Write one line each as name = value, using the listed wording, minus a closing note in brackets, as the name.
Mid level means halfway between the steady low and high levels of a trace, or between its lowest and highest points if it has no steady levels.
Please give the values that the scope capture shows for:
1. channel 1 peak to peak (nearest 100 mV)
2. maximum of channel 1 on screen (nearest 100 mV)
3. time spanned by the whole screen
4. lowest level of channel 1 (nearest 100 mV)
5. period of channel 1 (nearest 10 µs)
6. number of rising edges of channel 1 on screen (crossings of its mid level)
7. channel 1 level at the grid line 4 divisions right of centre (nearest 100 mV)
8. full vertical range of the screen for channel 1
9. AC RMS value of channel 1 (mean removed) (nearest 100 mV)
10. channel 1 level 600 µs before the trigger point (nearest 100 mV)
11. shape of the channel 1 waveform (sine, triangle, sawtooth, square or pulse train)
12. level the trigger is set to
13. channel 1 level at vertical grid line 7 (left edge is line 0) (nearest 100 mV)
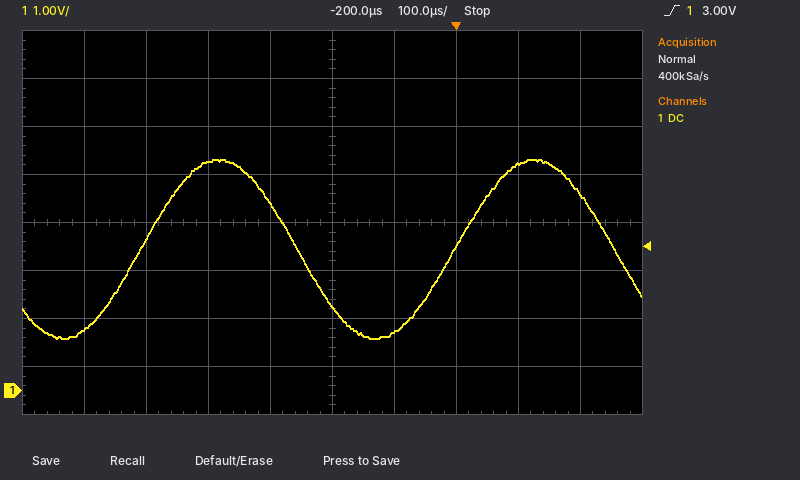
channel 1 peak to peak = 3.7 V
maximum of channel 1 on screen = 4.8 V
time spanned by the whole screen = 1 ms
lowest level of channel 1 = 1.1 V
period of channel 1 = 510 µs
number of rising edges of channel 1 on screen = 2
channel 1 level at the grid line 4 divisions right of centre = 4.1 V
full vertical range of the screen for channel 1 = 8 V
AC RMS value of channel 1 (mean removed) = 1.3 V
channel 1 level 600 µs before the trigger point = 1.3 V
shape of the channel 1 waveform = sine
level the trigger is set to = 3.00 V
channel 1 level at vertical grid line 7 (left edge is line 0) = 3.0 V
